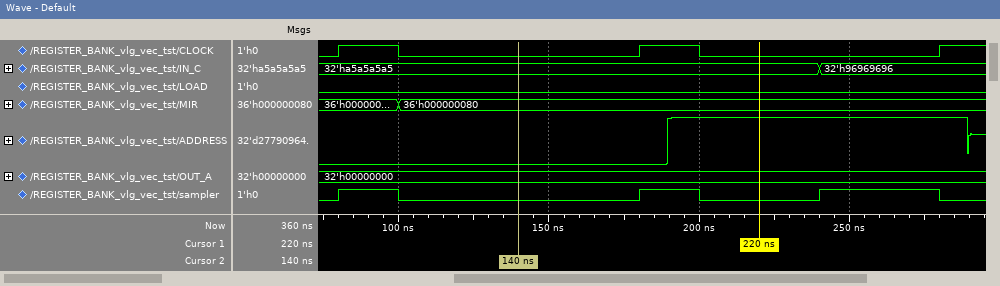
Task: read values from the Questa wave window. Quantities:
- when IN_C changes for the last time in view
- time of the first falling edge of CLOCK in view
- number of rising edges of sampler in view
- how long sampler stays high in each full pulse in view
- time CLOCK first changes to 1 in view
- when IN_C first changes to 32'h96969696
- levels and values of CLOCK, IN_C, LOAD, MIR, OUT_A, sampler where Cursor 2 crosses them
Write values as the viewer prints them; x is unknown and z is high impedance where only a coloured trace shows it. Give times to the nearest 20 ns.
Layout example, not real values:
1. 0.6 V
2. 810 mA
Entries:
1. 240 ns
2. 100 ns
3. 3
4. 20 ns, 20 ns, 40 ns
5. 80 ns
6. 240 ns
7. CLOCK=0, IN_C=32'ha5a5a5a5, LOAD=0, MIR=36'h000000080, OUT_A=32'h00000000, sampler=0
